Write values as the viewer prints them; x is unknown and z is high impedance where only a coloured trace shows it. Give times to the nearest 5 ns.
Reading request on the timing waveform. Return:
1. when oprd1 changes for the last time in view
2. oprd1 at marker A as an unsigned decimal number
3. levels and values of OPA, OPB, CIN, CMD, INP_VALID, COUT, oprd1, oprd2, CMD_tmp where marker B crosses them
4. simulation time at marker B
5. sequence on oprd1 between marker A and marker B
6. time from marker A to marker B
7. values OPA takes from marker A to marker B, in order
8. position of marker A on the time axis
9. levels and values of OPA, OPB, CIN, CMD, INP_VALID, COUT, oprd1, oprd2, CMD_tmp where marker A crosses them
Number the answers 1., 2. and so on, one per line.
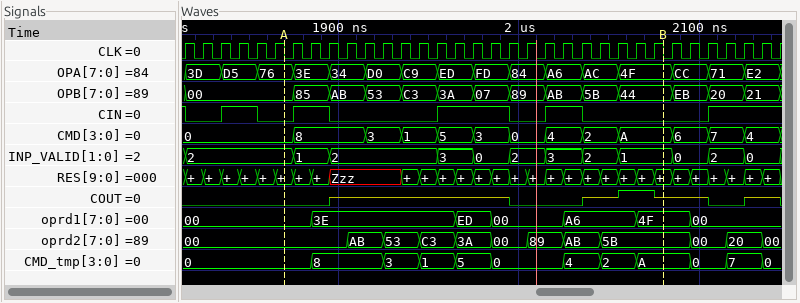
1. 2095 ns
2. 0
3. OPA=4F, OPB=44, CIN=0, CMD=A, INP_VALID=1, COUT=z, oprd1=4F, oprd2=5B, CMD_tmp=A
4. 2080 ns
5. 00, 3E, ED, 00, A6, 4F
6. 210 ns
7. 76, 3E, 34, D0, C9, ED, FD, 84, A6, AC, 4F
8. 1870 ns
9. OPA=76, OPB=00, CIN=0, CMD=0, INP_VALID=2, COUT=0, oprd1=00, oprd2=00, CMD_tmp=0
